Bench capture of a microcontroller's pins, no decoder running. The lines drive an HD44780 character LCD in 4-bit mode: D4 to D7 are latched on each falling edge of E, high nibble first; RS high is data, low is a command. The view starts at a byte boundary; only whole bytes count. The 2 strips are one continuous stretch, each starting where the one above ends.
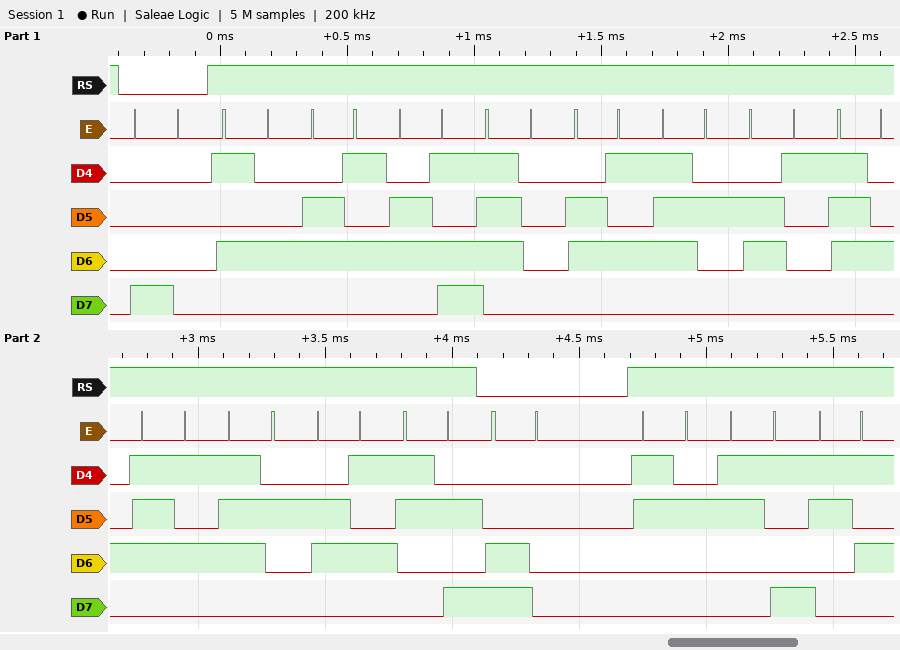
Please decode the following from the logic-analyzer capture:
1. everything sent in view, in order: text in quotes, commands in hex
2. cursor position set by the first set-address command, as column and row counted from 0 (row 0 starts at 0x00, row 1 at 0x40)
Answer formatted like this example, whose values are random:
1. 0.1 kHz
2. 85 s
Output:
1. 0x80 "Temperature:" 0xC0 "295"
2. column 0, row 0
